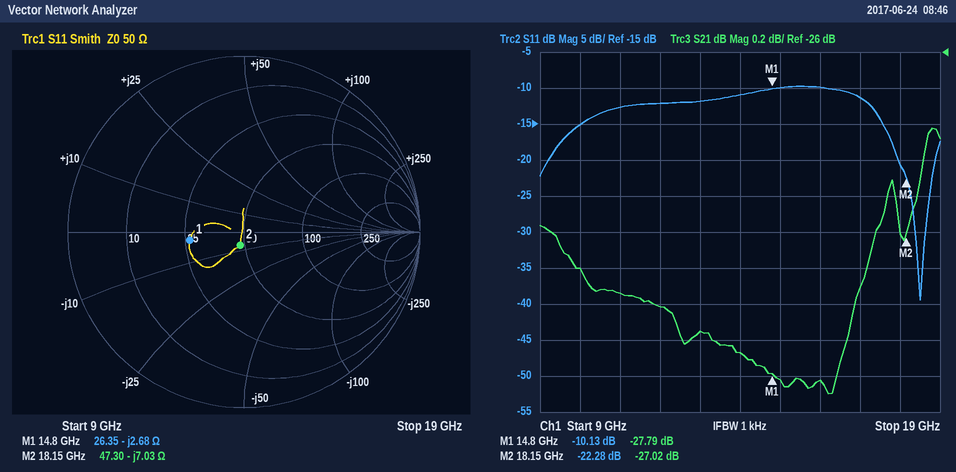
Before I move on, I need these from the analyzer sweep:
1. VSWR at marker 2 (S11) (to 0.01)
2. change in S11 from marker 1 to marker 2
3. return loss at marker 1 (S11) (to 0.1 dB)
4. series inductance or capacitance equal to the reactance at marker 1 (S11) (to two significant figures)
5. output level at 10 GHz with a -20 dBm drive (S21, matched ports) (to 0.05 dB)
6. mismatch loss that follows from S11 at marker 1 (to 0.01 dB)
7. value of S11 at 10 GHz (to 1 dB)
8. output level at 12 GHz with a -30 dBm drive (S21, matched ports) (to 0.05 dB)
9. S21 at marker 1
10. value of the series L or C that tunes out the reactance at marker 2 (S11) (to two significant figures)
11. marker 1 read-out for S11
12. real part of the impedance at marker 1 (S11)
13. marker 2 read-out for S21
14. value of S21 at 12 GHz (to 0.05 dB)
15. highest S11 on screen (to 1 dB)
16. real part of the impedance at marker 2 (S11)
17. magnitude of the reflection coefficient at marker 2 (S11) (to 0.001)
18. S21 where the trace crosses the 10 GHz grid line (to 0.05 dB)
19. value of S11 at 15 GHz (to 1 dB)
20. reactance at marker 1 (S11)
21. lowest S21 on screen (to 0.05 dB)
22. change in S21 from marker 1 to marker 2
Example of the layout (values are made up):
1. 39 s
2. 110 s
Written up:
1. 1.17
2. -12.15 dB
3. 10.1 dB
4. 4.0 pF
5. -47.20 dBm
6. 0.44 dB
7. -15 dB
8. -57.40 dBm
9. -27.79 dB
10. 62 pH
11. -10.13 dB
12. 26.35 Ω
13. -27.02 dB
14. -27.40 dB
15. -10 dB
16. 47.30 Ω
17. 0.077
18. -27.20 dB
19. -10 dB
20. -2.68 Ω
21. -27.90 dB
22. 0.77 dB
